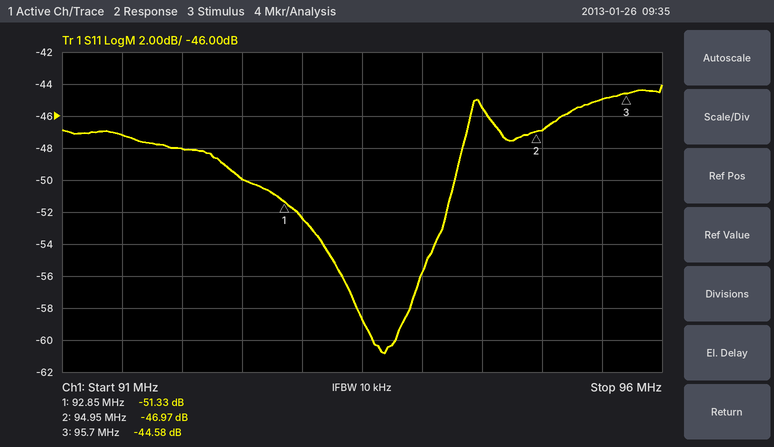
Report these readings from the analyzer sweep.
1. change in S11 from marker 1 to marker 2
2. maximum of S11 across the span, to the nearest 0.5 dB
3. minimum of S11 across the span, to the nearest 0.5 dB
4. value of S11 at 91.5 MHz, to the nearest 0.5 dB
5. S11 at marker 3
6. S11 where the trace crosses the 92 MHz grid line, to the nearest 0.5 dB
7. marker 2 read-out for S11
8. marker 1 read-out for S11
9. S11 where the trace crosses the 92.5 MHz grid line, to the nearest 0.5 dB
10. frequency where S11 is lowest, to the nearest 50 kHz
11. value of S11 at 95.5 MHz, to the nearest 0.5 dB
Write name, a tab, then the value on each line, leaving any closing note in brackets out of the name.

change in S11 from marker 1 to marker 2	4.36 dB
maximum of S11 across the span, to the nearest 0.5 dB	-44.0 dB
minimum of S11 across the span, to the nearest 0.5 dB	-61.0 dB
value of S11 at 91.5 MHz, to the nearest 0.5 dB	-47.0 dB
S11 at marker 3	-44.58 dB
S11 where the trace crosses the 92 MHz grid line, to the nearest 0.5 dB	-48.0 dB
marker 2 read-out for S11	-46.97 dB
marker 1 read-out for S11	-51.33 dB
S11 where the trace crosses the 92.5 MHz grid line, to the nearest 0.5 dB	-50.0 dB
frequency where S11 is lowest, to the nearest 50 kHz	93.70 MHz
value of S11 at 95.5 MHz, to the nearest 0.5 dB	-45.0 dB
